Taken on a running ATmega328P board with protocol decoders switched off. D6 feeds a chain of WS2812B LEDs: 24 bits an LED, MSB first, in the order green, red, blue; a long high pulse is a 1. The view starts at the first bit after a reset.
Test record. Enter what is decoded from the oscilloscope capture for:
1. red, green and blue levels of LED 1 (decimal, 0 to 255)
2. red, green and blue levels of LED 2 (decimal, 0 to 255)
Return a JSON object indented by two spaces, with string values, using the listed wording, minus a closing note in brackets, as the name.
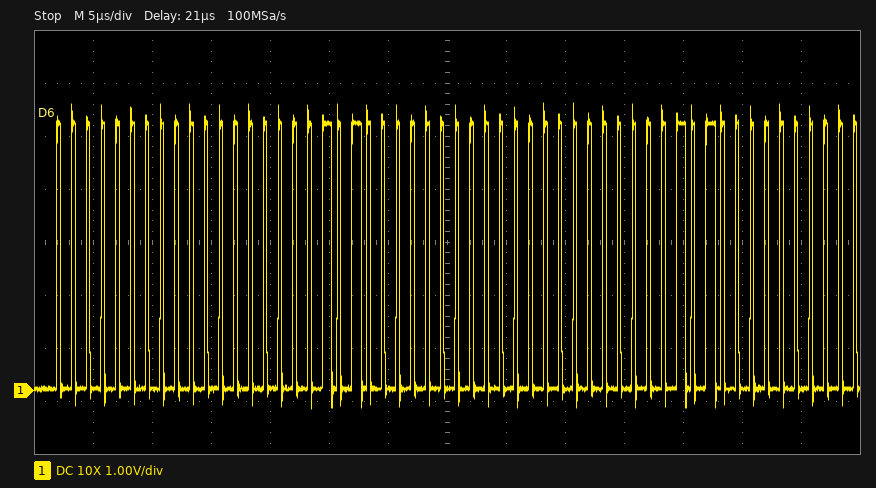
{
  "red, green and blue levels of LED 1": "0, 0, 40",
  "red, green and blue levels of LED 2": "0, 0, 40"
}
